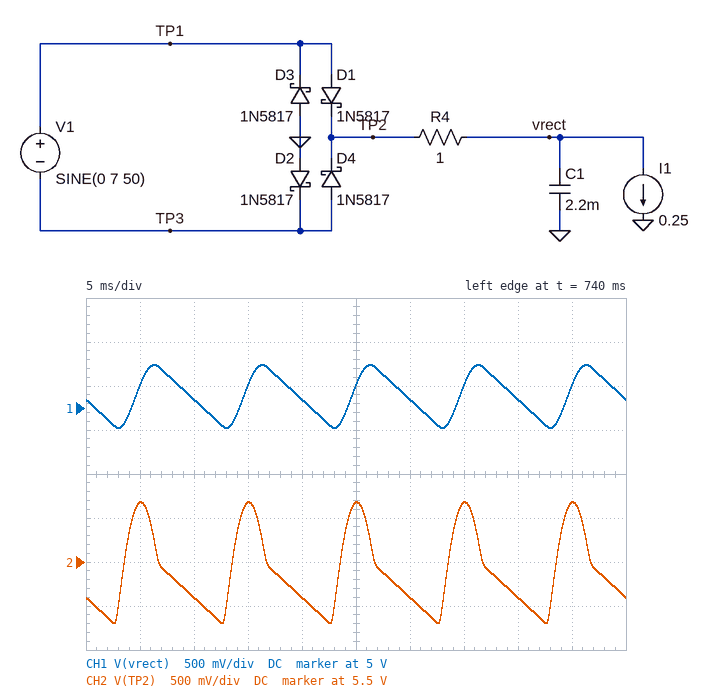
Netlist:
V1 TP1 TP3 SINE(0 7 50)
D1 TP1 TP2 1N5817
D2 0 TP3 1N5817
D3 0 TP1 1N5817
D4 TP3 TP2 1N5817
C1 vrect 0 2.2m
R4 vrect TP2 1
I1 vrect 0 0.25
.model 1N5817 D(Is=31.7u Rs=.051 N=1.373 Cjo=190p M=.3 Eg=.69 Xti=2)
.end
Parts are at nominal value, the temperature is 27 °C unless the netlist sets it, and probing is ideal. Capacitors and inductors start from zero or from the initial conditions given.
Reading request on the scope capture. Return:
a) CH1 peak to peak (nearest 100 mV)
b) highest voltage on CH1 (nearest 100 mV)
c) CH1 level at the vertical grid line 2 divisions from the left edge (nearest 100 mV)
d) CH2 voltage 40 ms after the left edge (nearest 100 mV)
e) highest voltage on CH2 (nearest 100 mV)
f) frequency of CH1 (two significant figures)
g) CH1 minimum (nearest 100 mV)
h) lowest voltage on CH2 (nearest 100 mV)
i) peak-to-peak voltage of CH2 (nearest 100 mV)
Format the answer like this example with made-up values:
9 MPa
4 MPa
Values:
700 mV
5.5 V
5.1 V
5.1 V
6.2 V
100 Hz
4.8 V
4.8 V
1.4 V
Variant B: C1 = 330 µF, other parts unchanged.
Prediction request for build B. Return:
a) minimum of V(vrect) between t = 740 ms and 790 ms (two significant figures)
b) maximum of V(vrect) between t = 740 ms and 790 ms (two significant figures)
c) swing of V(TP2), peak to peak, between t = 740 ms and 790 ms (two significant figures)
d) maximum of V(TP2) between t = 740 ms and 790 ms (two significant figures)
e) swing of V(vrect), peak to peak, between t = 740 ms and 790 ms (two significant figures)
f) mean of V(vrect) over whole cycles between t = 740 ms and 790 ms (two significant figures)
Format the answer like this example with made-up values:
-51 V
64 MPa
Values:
2.1 V
6.0 V
4.2 V
6.3 V
4.0 V
4.3 V
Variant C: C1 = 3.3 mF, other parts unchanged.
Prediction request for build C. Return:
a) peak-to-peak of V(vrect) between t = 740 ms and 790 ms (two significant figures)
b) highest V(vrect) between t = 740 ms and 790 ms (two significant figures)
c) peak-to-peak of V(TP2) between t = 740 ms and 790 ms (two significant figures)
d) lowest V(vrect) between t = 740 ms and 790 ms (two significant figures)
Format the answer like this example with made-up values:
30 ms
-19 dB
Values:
480 mV
5.4 V
1.2 V
4.9 V
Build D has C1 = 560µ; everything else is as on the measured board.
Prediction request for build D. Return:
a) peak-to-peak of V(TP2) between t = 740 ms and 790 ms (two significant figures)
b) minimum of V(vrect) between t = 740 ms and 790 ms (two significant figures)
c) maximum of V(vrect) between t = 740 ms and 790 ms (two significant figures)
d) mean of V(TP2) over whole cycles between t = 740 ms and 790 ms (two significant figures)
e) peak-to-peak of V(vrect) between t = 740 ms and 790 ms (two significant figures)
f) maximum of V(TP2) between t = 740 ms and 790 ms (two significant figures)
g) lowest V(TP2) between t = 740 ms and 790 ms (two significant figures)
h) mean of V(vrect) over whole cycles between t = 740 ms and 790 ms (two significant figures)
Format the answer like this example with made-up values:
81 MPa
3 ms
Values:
2.9 V
3.3 V
5.9 V
5.0 V
2.6 V
6.3 V
3.4 V
4.7 V
